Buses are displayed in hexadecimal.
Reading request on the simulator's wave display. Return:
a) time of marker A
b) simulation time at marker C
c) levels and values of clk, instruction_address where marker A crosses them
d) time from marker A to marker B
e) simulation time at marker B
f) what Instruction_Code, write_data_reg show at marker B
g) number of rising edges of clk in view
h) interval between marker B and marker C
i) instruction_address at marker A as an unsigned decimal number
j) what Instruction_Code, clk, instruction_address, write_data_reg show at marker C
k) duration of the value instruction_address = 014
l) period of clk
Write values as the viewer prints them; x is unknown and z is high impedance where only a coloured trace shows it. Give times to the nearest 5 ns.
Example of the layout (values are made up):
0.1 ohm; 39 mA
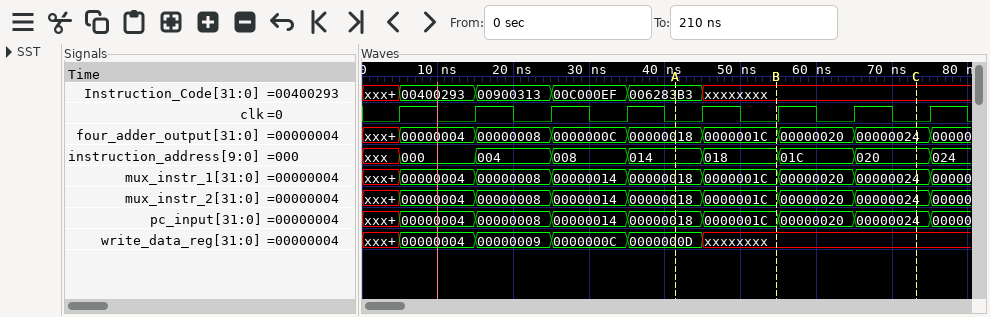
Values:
40 ns; 75 ns; clk=0, instruction_address=014; 15 ns; 55 ns; Instruction_Code=xxxxxxxx, write_data_reg=xxxxxxxx; 8; 20 ns; 20; Instruction_Code=xxxxxxxx, clk=0, instruction_address=020, write_data_reg=xxxxxxxx; 10 ns; 10 ns
